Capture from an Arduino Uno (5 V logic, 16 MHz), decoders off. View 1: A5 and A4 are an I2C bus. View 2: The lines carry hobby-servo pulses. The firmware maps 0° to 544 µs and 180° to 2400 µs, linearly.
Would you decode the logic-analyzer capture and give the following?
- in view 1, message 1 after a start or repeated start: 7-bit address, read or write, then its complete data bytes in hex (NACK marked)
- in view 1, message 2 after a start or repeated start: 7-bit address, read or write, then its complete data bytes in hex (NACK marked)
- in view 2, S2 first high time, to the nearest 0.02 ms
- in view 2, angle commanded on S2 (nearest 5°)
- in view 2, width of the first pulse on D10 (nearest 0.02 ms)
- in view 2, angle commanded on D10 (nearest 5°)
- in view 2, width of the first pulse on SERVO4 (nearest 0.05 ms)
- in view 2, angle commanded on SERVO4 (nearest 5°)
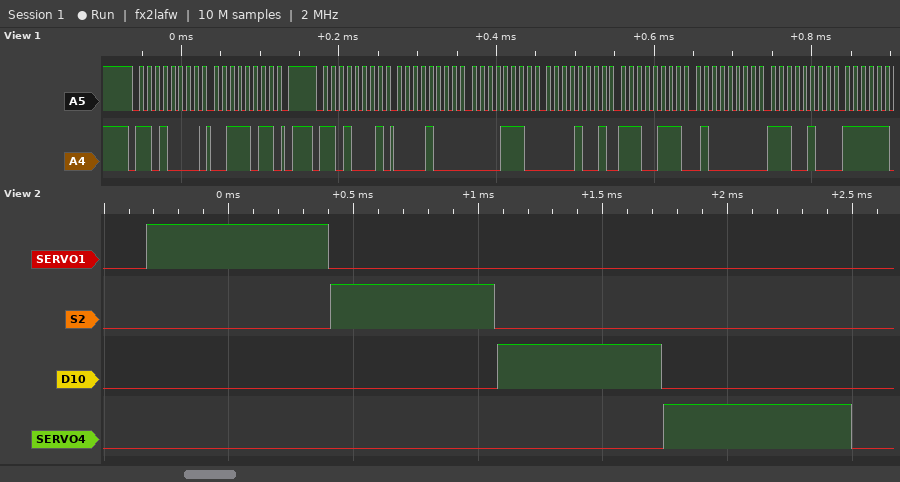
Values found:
0x68 write: 3B
0x68 read: 08 0E 09 E7 40 E4
0.66 ms
10°
0.66 ms
10°
0.75 ms
20°
